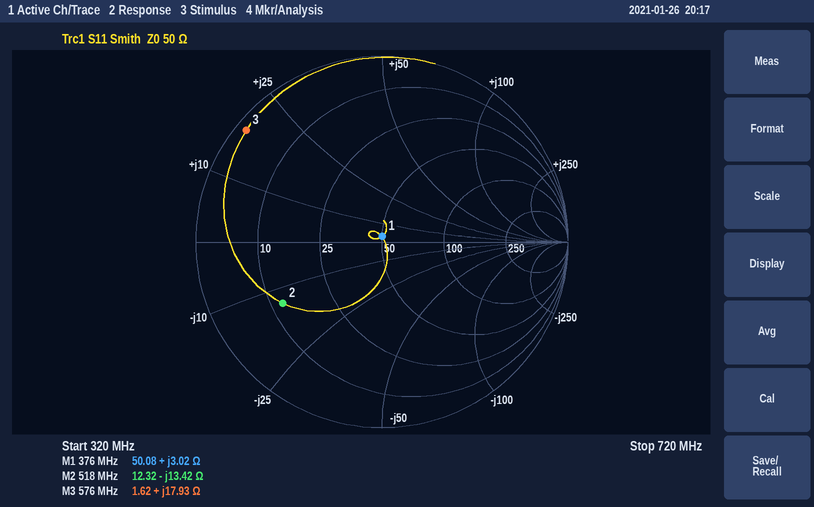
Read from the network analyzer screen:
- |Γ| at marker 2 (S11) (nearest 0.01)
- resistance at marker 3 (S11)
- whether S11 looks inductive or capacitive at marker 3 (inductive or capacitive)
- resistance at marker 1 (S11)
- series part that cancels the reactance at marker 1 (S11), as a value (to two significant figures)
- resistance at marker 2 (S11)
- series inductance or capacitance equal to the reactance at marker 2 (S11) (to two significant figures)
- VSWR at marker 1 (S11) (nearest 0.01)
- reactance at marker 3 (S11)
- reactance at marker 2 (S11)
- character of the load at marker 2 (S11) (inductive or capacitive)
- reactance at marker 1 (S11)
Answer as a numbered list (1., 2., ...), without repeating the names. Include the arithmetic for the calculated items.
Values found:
1. 0.63
2. 1.62 Ω
3. inductive
4. 50.08 Ω
5. C = 1/(2π × 376 MHz × 3.02 Ω) ≈ 140 pF
6. 12.32 Ω
7. C = 1/(2π × 518 MHz × 13.42 Ω) ≈ 23 pF
8. 1.06
9. +17.93 Ω
10. -13.42 Ω
11. capacitive
12. +3.02 Ω
